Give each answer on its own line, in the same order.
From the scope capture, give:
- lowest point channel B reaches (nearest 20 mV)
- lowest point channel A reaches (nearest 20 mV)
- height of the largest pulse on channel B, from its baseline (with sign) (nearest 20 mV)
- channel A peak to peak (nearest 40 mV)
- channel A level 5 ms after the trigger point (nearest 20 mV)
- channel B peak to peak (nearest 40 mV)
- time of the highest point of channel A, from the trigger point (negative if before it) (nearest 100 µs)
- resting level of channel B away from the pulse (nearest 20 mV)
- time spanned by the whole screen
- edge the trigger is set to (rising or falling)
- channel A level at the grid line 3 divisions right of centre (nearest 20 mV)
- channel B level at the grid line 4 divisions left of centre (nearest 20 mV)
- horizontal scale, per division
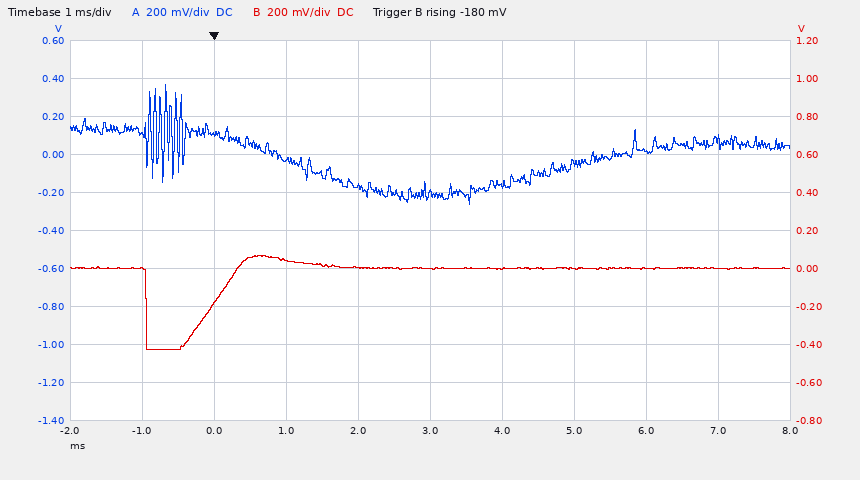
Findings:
-420 mV
-260 mV
-420 mV
640 mV
-40 mV
480 mV
-700 µs
0 mV
10 ms
rising
20 mV
0 mV
1 ms
